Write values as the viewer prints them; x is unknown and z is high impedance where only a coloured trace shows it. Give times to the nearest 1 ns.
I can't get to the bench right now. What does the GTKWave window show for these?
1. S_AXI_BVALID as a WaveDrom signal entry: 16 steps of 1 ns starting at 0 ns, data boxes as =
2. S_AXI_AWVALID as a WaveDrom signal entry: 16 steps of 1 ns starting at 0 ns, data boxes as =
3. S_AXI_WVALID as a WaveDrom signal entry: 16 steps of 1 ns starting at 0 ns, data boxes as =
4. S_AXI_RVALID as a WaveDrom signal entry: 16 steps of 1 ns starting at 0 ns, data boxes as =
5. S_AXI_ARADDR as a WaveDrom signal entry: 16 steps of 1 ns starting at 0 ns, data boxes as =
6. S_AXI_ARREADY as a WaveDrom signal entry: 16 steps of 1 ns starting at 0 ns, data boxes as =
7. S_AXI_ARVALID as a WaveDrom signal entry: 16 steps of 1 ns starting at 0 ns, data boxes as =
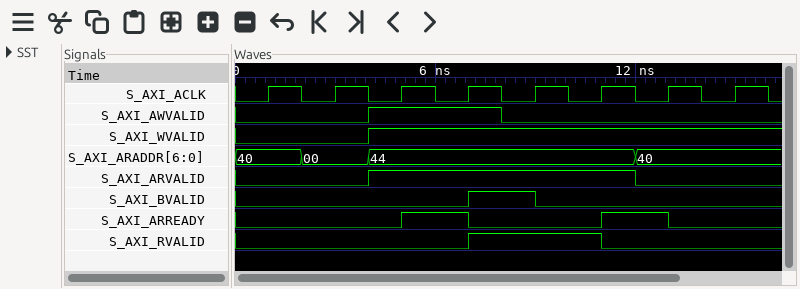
{name: 'S_AXI_BVALID', wave: '0......1.0......'}
{name: 'S_AXI_AWVALID', wave: '0...1...0.......'}
{name: 'S_AXI_WVALID', wave: '0...1...........'}
{name: 'S_AXI_RVALID', wave: '0......1...0....'}
{name: 'S_AXI_ARADDR', wave: '=.=.=.......=...', data: '40 00 44 40'}
{name: 'S_AXI_ARREADY', wave: '0....1.0...1.0..'}
{name: 'S_AXI_ARVALID', wave: '0...1.......0...'}
